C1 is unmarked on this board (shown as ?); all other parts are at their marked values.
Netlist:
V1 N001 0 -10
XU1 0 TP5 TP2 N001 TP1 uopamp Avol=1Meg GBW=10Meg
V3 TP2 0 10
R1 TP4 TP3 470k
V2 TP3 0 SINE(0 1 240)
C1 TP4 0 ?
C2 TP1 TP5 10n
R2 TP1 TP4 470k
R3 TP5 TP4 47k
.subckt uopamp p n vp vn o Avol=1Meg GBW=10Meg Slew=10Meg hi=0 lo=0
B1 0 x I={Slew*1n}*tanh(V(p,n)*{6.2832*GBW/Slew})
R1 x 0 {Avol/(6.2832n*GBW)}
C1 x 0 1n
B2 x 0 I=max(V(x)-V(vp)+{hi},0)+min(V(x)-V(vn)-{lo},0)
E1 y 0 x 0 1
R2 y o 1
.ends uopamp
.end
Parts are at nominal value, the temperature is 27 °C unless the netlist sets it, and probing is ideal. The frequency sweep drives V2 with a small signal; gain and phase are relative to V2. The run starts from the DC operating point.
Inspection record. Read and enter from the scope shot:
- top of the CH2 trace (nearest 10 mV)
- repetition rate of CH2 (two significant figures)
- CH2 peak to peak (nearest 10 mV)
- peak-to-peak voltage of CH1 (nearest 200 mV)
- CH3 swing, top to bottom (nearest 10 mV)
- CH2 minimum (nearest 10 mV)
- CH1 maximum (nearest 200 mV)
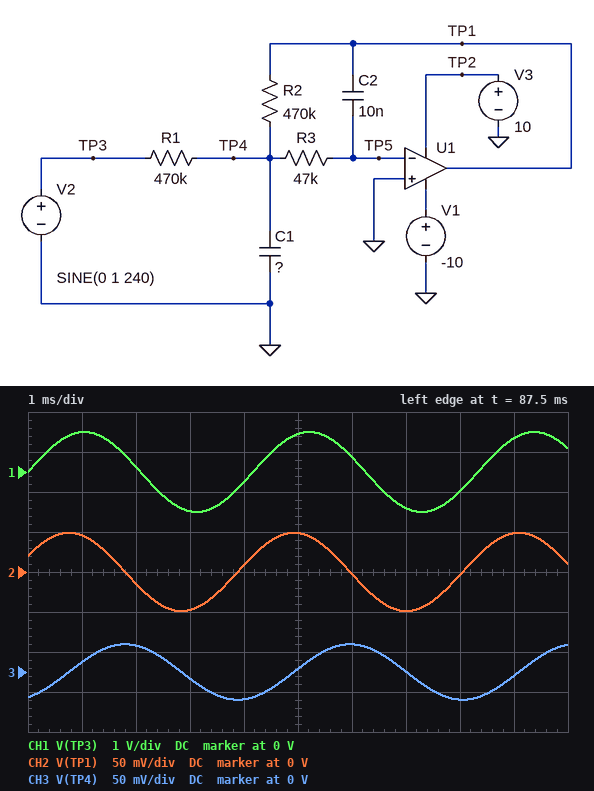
50 mV
240 Hz
100 mV
2.0 V
70 mV
-50 mV
1.0 V
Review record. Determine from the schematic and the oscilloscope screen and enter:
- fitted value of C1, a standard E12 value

39 nF
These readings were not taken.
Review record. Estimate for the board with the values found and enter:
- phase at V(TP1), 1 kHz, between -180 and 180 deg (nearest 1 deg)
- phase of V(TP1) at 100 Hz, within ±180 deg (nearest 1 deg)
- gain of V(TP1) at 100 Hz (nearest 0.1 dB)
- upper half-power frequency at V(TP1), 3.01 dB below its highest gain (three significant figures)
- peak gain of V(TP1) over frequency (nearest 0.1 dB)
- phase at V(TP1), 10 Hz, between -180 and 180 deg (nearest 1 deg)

6 deg
56 deg
-12.6 dB
36.9 Hz
0 dB
160 deg
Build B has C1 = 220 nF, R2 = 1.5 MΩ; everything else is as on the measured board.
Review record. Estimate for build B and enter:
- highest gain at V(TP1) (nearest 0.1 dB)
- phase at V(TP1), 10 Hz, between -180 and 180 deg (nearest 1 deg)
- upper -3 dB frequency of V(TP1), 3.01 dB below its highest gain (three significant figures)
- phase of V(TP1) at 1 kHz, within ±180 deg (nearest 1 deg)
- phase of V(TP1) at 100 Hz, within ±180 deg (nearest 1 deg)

10.1 dB
110 deg
13.2 Hz
1 deg
10 deg
